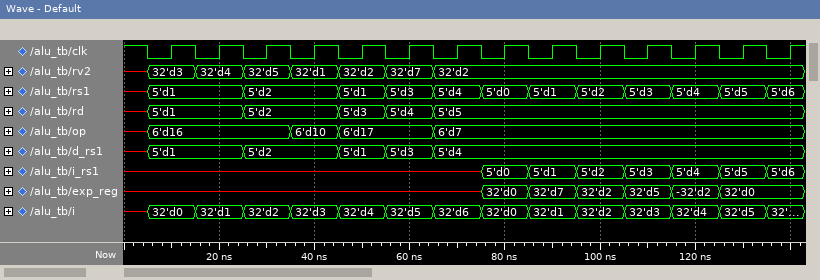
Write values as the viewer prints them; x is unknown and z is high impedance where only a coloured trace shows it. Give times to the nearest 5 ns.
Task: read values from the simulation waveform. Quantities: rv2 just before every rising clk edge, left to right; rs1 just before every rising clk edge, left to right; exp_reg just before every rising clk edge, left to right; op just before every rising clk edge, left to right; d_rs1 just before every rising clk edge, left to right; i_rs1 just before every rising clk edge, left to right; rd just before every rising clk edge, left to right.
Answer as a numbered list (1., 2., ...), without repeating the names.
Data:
1. 32'd3, 32'd4, 32'd5, 32'd1, 32'd2, 32'd7, 32'd2, 32'd2, 32'd2, 32'd2, 32'd2, 32'd2, 32'd2, 32'd2
2. 5'd1, 5'd1, 5'd2, 5'd2, 5'd1, 5'd3, 5'd4, 5'd0, 5'd1, 5'd2, 5'd3, 5'd4, 5'd5, 5'd6
3. x, x, x, x, x, x, x, 32'd0, 32'd7, 32'd2, 32'd5, -32'd2, 32'd0, 32'd0
4. 6'd16, 6'd16, 6'd16, 6'd10, 6'd17, 6'd17, 6'd7, 6'd7, 6'd7, 6'd7, 6'd7, 6'd7, 6'd7, 6'd7
5. 5'd1, 5'd1, 5'd2, 5'd2, 5'd1, 5'd3, 5'd4, 5'd4, 5'd4, 5'd4, 5'd4, 5'd4, 5'd4, 5'd4
6. x, x, x, x, x, x, x, 5'd0, 5'd1, 5'd2, 5'd3, 5'd4, 5'd5, 5'd6
7. 5'd1, 5'd1, 5'd2, 5'd2, 5'd3, 5'd4, 5'd5, 5'd5, 5'd5, 5'd5, 5'd5, 5'd5, 5'd5, 5'd5
